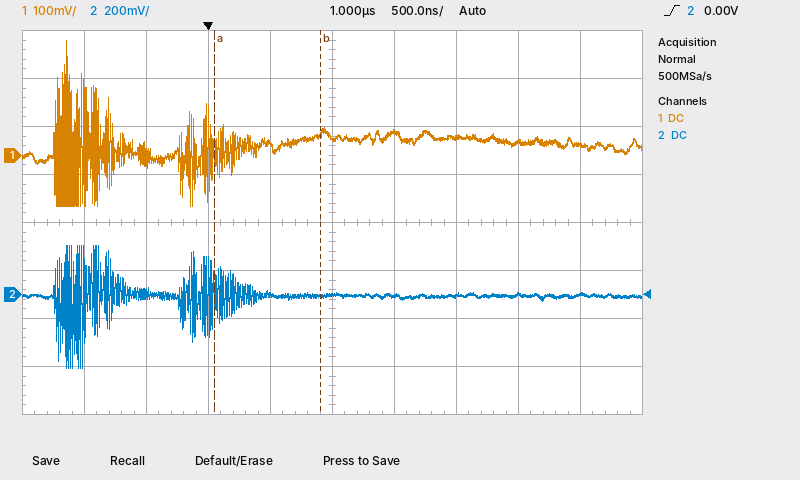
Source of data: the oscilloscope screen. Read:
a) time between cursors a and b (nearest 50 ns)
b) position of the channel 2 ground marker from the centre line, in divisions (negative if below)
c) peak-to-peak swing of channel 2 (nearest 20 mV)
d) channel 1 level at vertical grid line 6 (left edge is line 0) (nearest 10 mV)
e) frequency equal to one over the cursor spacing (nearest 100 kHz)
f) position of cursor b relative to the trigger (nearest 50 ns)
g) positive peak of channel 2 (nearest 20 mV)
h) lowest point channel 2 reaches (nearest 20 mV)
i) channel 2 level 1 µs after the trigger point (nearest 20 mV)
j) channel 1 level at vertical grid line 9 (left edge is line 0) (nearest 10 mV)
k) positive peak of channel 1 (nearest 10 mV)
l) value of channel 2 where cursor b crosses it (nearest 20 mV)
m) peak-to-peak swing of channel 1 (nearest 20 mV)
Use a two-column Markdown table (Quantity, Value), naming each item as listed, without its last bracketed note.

| Quantity | Value |
|---|---|
| time between cursors a and b | 850 ns |
| position of the channel 2 ground marker from the centre line, in divisions | -1.5 div |
| peak-to-peak swing of channel 2 | 500 mV |
| channel 1 level at vertical grid line 6 (left edge is line 0) | 50 mV |
| frequency equal to one over the cursor spacing | 1.2 MHz |
| position of cursor b relative to the trigger | +900 ns |
| positive peak of channel 2 | 200 mV |
| lowest point channel 2 reaches | -300 mV |
| channel 2 level 1 µs after the trigger point | 0 mV |
| channel 1 level at vertical grid line 9 (left edge is line 0) | 20 mV |
| positive peak of channel 1 | 240 mV |
| value of channel 2 where cursor b crosses it | 0 mV |
| peak-to-peak swing of channel 1 | 340 mV |
